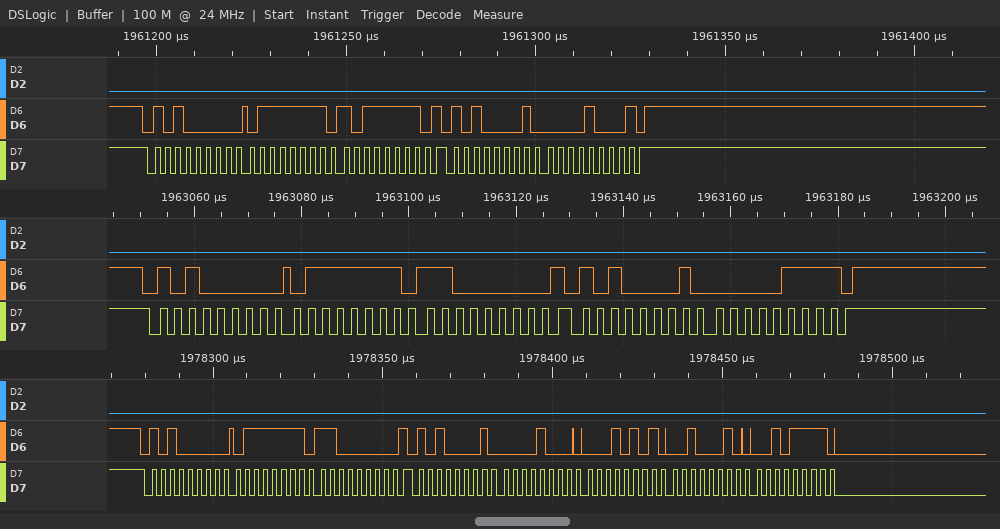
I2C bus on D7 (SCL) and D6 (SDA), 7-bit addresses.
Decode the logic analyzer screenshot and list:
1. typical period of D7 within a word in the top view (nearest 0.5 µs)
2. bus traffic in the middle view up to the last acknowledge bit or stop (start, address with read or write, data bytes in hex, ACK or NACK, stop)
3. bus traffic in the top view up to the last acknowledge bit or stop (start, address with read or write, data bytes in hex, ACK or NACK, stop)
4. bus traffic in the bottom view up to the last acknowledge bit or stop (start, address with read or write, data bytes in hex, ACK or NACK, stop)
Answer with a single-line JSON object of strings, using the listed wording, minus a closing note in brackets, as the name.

{"typical period of D7 within a word in the top view": "2.5 µs", "bus traffic in the middle view up to the last acknowledge bit or stop": "start, address 50 write ACK, 7F ACK, C0 ACK, repeated start, address 50 read ACK, 07 NACK, stop", "bus traffic in the top view up to the last acknowledge bit or stop": "start, address 50 write ACK, 7F ACK, BF ACK, repeated start, address 50 read ACK, 08 NACK, stop", "bus traffic in the bottom view up to the last acknowledge bit or stop": "start, address 50 write ACK, 7F ACK, C0 ACK, repeated start, address 50 read ACK, 08 ACK, 15 ACK, 22 ACK, 2F ACK"}
